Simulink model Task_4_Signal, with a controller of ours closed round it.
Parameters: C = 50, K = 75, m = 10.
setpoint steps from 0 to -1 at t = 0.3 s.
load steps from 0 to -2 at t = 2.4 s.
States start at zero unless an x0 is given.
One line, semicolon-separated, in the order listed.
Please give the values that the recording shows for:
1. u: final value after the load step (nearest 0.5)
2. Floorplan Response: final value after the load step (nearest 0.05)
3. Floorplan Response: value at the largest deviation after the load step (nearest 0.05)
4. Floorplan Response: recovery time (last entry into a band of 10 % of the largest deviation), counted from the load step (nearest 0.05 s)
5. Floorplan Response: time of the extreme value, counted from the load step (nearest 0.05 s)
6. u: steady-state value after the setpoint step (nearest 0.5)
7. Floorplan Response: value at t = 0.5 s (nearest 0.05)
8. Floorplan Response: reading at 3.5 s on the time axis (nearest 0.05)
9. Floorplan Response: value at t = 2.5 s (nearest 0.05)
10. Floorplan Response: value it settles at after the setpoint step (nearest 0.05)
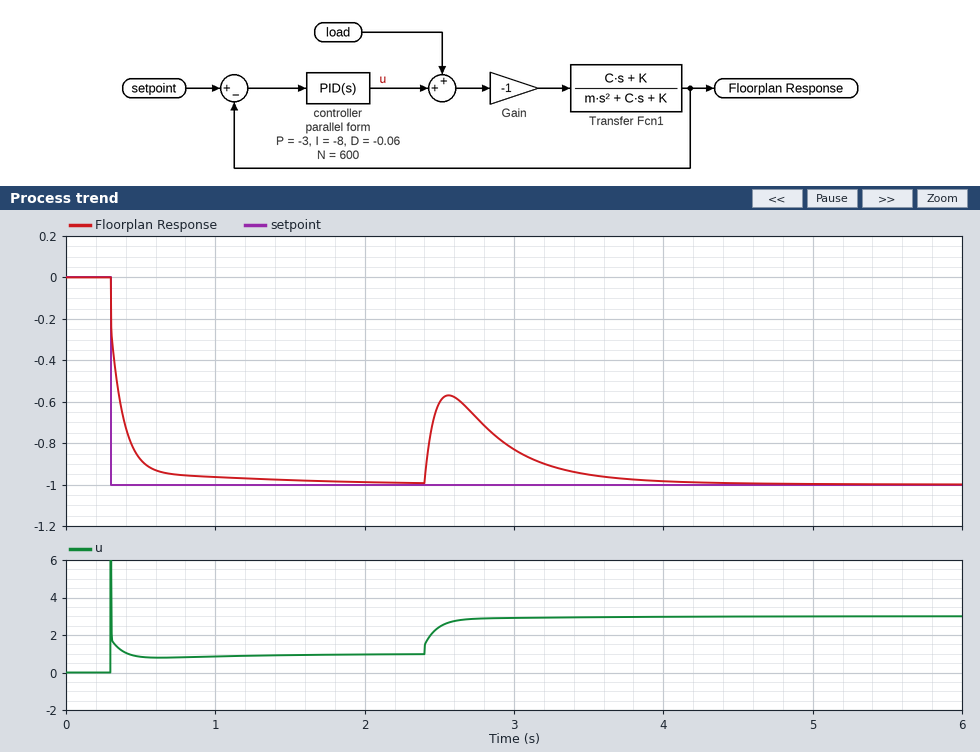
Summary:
3.0; -1.00; -0.55; 1.15 s; 0.15 s; 1.0; -0.90; -0.95; -0.60; -1.00
